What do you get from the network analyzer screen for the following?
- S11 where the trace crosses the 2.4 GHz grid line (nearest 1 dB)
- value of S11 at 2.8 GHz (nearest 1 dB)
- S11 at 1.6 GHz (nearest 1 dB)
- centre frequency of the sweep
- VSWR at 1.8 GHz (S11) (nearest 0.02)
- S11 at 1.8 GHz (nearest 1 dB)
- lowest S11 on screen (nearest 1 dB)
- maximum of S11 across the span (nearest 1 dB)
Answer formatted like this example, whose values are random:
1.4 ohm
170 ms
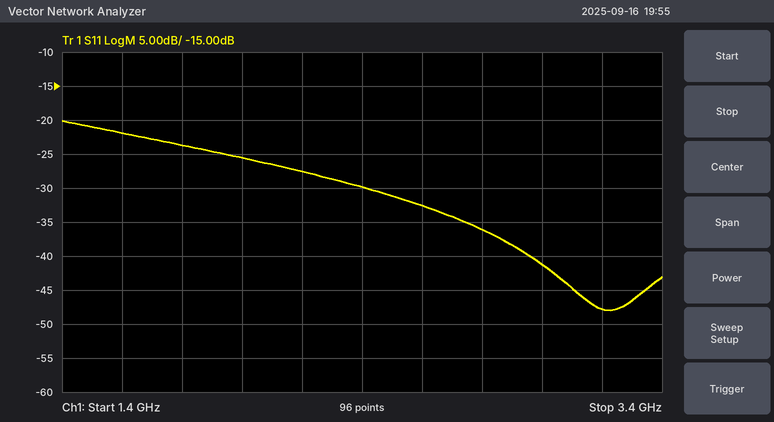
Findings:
-30 dB
-36 dB
-22 dB
2.4 GHz
1.14
-24 dB
-48 dB
-20 dB
